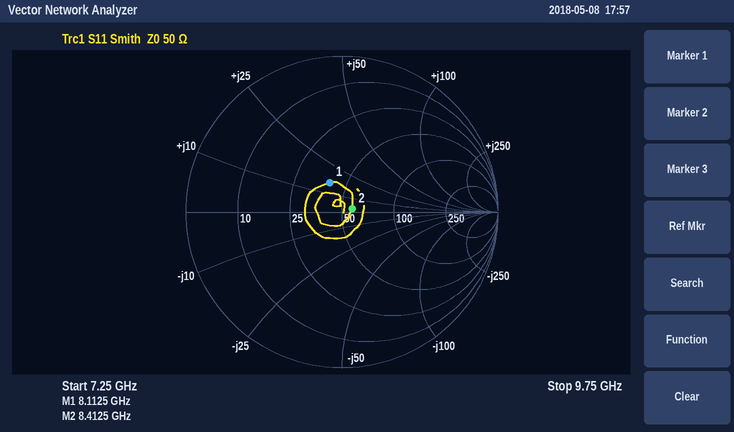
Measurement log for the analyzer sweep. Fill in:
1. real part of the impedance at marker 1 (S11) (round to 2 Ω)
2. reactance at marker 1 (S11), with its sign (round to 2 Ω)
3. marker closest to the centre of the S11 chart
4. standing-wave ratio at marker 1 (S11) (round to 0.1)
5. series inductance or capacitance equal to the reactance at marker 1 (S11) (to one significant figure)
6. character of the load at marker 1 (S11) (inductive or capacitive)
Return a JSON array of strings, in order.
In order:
["40 Ω", "+16 Ω", "marker 2", "1.5", "300 pH", "inductive"]
